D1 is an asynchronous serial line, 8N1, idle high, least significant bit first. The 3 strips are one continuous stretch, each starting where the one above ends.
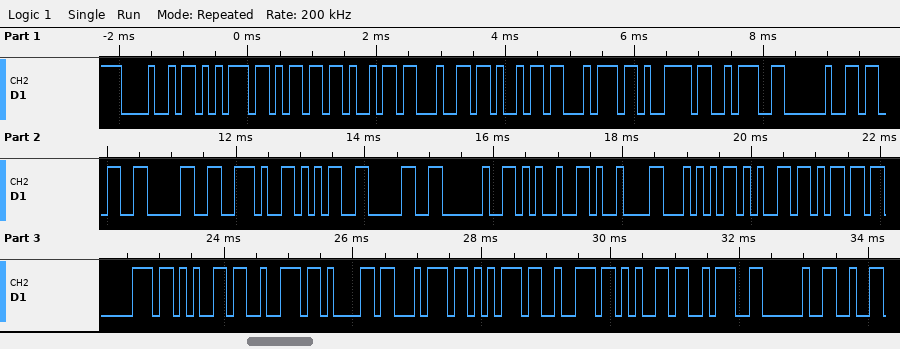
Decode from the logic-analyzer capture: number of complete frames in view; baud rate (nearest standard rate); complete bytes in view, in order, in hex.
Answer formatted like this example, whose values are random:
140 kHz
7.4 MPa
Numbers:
31
9600 baud
48 75 6D 69 64 69 74 79 3A 20 33 30 2E 35 30 20 25 09 54 65 6D 70 65 72 61 74 75 72 65 3A 20
